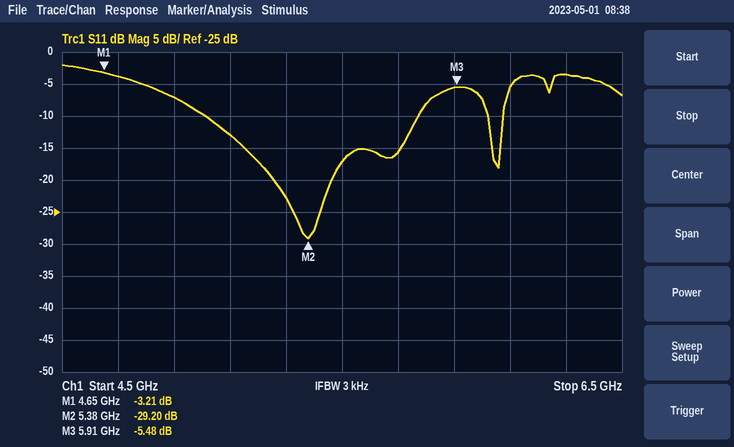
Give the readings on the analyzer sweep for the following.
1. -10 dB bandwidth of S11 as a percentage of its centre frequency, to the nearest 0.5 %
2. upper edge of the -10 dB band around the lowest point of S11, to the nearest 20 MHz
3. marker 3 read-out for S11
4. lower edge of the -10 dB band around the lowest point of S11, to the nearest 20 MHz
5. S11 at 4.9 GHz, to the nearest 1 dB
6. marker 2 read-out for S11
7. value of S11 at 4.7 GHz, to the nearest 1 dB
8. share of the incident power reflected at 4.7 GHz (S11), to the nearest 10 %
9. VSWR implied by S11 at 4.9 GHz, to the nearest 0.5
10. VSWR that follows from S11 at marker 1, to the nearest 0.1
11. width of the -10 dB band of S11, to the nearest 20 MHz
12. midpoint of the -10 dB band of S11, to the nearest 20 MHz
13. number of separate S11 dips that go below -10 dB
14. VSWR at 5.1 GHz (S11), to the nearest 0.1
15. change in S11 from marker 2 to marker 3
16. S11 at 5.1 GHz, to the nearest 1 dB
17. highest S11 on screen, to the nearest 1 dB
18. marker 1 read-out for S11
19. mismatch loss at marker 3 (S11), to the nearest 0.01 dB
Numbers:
14.0 %
5.78 GHz
-5.48 dB
5.02 GHz
-7 dB
-29.20 dB
-4 dB
40 %
2.5
5.5
760 MHz
5.40 GHz
2
1.6
23.72 dB
-13 dB
-2 dB
-3.21 dB
1.45 dB
